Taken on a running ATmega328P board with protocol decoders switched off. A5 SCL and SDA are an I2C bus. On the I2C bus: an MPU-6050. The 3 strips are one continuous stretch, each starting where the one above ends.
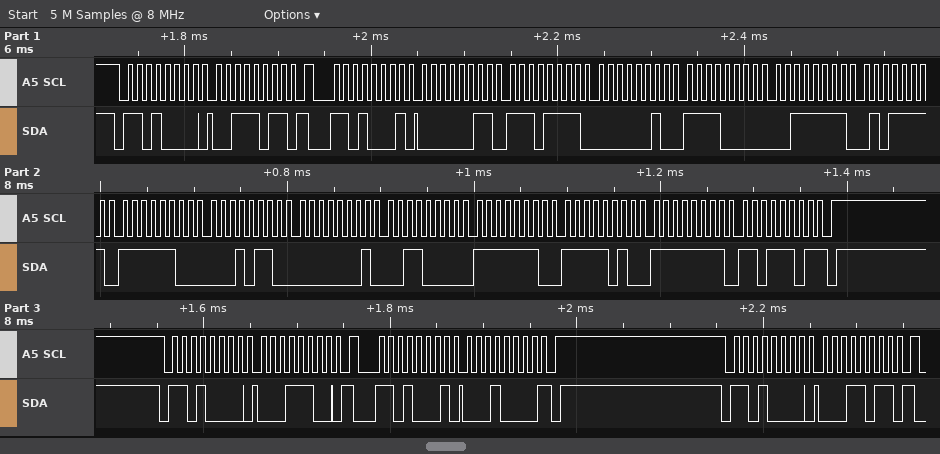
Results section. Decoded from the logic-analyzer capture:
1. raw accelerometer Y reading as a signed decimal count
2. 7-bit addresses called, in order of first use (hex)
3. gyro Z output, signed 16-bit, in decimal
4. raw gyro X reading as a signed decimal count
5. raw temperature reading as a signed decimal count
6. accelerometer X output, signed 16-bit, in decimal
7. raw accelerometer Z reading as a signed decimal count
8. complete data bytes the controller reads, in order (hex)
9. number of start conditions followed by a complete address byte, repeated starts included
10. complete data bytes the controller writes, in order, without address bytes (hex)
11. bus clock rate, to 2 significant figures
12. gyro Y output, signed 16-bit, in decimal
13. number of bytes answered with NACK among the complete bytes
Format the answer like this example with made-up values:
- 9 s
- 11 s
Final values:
- 752
- 0x68
- -35
- 304
- -1002
- 1007
- 16223
- 03 EF 02 F0 3F 5F FC 16 01 30 FE FA FF DD 10
- 5
- 3B 1C 1B
- 100 kHz
- -262
- 2
